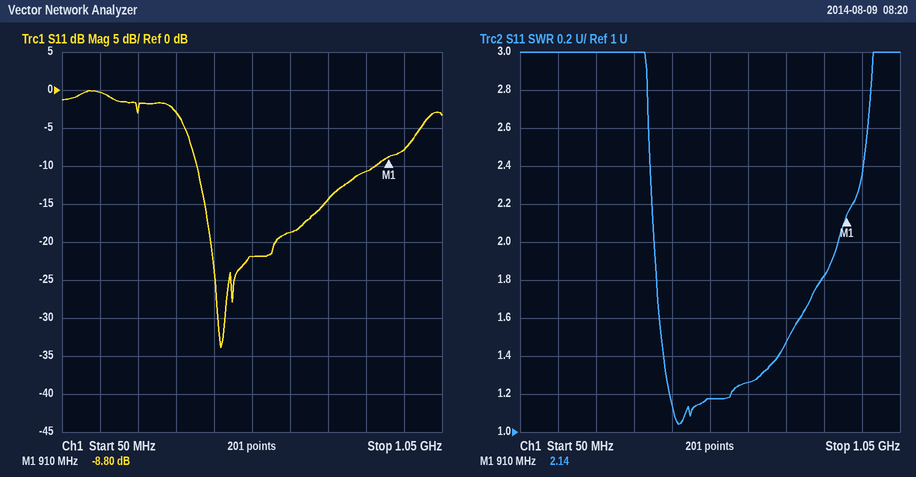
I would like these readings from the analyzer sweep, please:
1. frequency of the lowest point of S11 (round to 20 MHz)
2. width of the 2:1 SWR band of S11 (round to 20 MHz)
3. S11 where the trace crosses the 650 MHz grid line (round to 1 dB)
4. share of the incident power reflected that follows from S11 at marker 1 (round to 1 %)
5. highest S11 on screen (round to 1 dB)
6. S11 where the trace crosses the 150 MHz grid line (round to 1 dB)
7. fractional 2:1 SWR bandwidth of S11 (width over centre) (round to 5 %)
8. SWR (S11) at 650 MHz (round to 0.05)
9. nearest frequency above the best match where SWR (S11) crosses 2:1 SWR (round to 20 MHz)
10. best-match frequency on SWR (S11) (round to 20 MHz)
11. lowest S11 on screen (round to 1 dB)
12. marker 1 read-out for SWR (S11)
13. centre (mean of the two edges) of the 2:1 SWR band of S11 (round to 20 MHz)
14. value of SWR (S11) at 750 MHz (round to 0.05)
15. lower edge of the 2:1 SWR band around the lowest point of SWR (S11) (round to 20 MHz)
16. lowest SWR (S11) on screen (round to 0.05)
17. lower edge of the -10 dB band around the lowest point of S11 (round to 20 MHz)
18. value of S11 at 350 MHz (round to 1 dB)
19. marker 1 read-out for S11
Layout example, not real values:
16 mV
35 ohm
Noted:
460 MHz
480 MHz
-19 dB
13 %
0 dB
0 dB
75 %
1.25
880 MHz
460 MHz
-34 dB
2.14
640 MHz
1.45
400 MHz
1.05
400 MHz
-3 dB
-8.80 dB
